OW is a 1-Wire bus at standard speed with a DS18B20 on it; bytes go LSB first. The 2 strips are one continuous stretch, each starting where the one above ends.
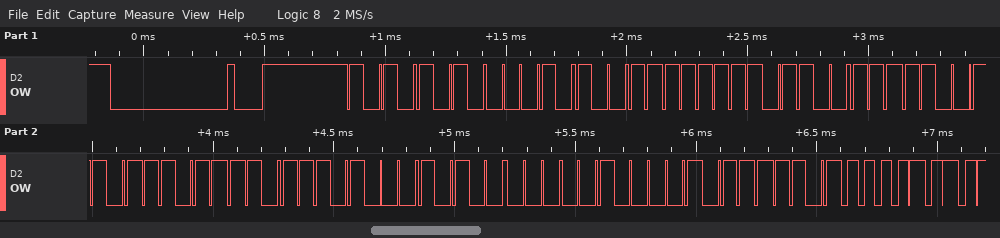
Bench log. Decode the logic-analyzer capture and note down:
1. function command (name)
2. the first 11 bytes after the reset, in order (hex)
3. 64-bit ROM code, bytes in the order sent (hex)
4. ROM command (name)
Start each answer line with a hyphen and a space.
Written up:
- Read Scratchpad
- 55 28 FF E6 B3 7B 17 05 84 BE 50
- 28 FF E6 B3 7B 17 05 84
- Match ROM
